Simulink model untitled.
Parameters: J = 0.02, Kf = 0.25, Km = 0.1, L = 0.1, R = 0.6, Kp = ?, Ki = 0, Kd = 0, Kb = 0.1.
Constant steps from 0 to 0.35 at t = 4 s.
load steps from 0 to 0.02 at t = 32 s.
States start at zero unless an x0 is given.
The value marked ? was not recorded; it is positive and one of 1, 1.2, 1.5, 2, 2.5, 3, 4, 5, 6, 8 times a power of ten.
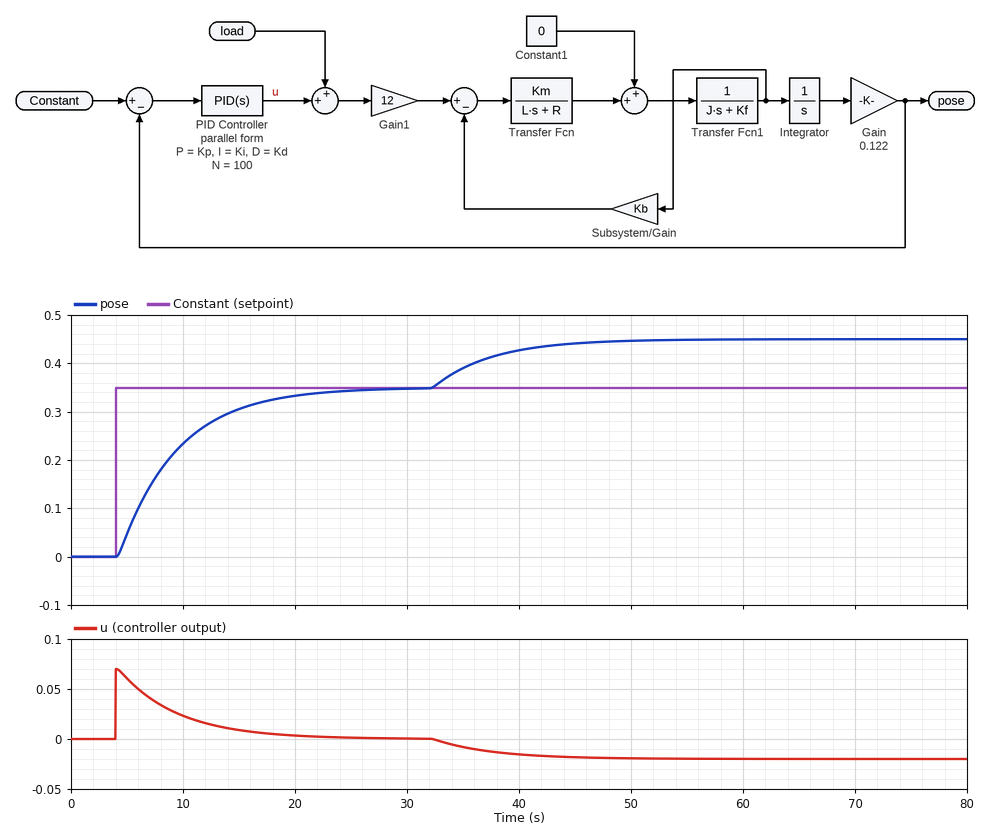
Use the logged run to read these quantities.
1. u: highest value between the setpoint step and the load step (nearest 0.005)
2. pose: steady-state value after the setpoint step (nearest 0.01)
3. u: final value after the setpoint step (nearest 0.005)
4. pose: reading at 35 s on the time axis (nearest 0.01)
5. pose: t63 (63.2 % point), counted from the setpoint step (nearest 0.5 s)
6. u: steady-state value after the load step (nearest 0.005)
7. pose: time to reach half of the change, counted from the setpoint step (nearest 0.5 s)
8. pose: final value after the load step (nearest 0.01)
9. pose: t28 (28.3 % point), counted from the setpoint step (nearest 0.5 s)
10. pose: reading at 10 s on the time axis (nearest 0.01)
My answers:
0.070
0.35
0.000
0.39
5.5 s
-0.020
4.0 s
0.45
2.0 s
0.23
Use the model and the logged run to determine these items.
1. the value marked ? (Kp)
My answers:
0.2
